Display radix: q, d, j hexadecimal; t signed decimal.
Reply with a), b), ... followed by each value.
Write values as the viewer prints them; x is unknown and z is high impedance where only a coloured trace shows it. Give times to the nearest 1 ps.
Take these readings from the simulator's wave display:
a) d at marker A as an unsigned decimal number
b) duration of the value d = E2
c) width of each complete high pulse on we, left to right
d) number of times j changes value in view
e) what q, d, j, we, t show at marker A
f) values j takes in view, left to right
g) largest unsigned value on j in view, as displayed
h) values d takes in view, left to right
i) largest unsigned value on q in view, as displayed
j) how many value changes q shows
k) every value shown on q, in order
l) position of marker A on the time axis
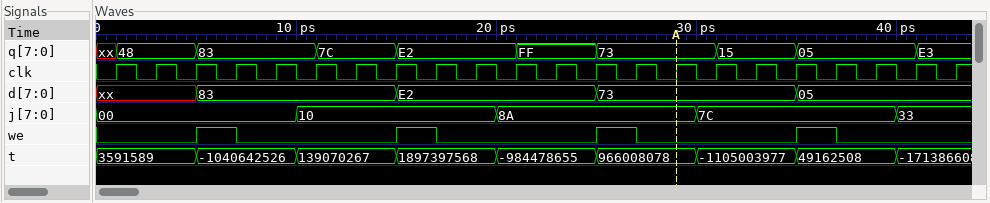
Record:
a) 115
b) 10 ps
c) 2 ps, 2 ps, 2 ps, 2 ps
d) 4
e) q=73, d=73, j=8A, we=0, t=966008078
f) 00, 10, 8A, 7C, 33
g) 8A
h) xx, 83, E2, 73, 05
i) FF
j) 9
k) xx, 48, 83, 7C, E2, FF, 73, 15, 05, E3
l) 29 ps
